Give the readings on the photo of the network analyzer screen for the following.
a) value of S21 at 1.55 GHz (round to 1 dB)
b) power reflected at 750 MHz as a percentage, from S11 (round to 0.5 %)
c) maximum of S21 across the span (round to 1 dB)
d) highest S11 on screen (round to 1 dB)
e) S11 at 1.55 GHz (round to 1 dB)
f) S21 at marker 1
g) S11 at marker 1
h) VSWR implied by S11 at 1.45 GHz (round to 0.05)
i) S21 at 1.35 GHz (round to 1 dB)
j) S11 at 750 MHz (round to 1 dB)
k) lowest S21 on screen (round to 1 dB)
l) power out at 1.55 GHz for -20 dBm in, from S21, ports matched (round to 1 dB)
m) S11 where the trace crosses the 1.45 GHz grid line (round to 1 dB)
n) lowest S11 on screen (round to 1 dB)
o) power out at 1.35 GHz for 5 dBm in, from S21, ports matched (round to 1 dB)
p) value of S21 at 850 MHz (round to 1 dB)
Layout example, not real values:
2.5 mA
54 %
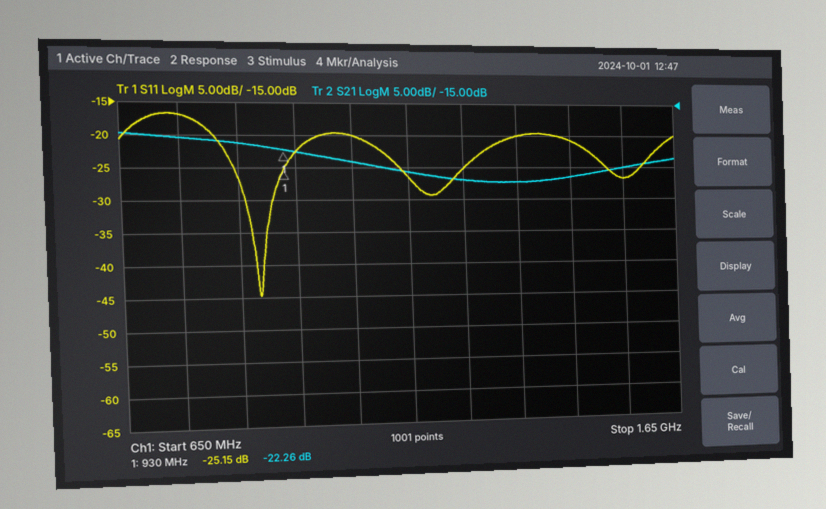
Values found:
-25 dB
2.0 %
-20 dB
-17 dB
-27 dB
-22.26 dB
-25.15 dB
1.20
-27 dB
-17 dB
-27 dB
-45 dBm
-21 dB
-45 dB
-22 dBm
-21 dB
